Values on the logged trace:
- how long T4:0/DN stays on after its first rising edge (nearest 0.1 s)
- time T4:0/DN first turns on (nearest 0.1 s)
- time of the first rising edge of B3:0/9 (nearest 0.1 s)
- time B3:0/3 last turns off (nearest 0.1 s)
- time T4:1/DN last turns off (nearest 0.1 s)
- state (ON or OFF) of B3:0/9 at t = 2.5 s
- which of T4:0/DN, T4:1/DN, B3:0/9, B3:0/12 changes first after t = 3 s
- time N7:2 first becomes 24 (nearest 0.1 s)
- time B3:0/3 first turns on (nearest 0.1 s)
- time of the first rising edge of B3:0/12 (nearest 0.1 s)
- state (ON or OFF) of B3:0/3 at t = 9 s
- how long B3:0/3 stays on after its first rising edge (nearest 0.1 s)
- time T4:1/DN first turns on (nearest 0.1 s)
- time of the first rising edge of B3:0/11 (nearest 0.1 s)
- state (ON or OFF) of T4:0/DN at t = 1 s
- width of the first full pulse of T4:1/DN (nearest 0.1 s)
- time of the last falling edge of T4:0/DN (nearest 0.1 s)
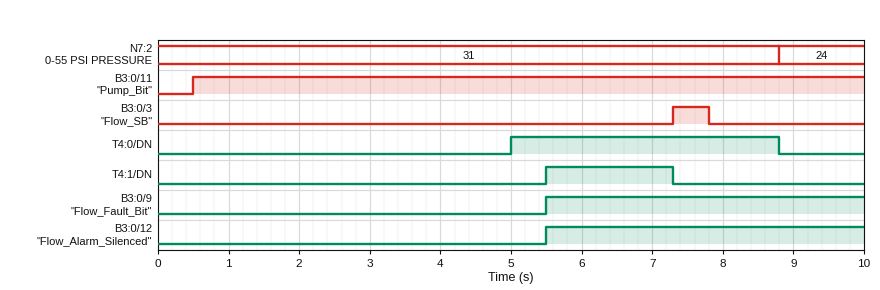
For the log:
3.8 s
5.0 s
5.5 s
7.8 s
7.3 s
OFF
T4:0/DN
8.8 s
7.3 s
5.5 s
OFF
0.5 s
5.5 s
0.5 s
OFF
1.8 s
8.8 s
